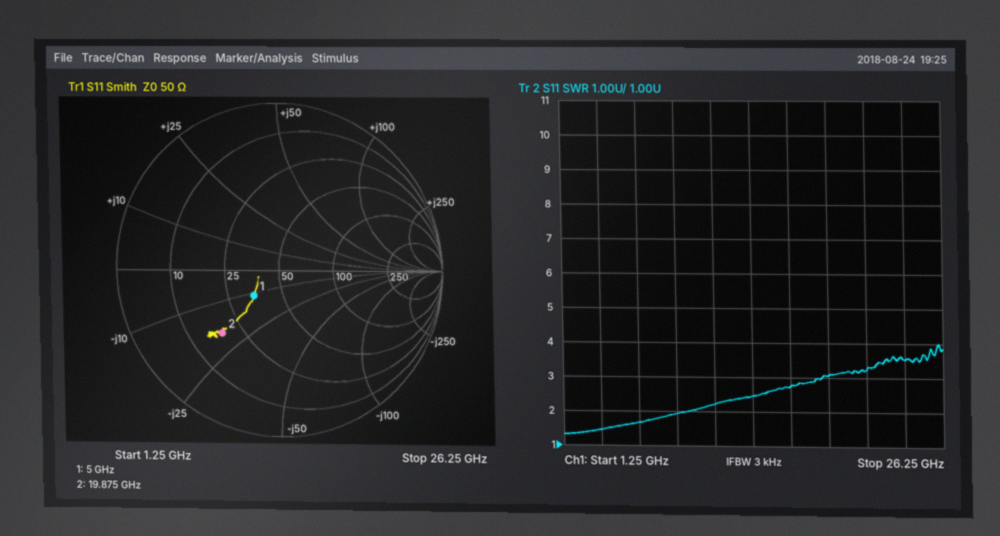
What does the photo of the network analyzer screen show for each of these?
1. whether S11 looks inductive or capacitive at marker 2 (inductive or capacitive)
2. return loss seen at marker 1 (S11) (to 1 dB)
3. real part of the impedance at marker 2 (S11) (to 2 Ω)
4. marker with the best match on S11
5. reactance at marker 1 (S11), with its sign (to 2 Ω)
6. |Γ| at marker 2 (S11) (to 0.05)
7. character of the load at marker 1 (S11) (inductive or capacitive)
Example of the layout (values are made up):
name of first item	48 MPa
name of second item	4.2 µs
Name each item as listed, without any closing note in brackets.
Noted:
whether S11 looks inductive or capacitive at marker 2	capacitive
return loss seen at marker 1 (S11)	13 dB
real part of the impedance at marker 2 (S11)	18 Ω
marker with the best match on S11	marker 1
reactance at marker 1 (S11), with its sign	-12 Ω
|Γ| at marker 2 (S11)	0.50
character of the load at marker 1 (S11)	capacitive
